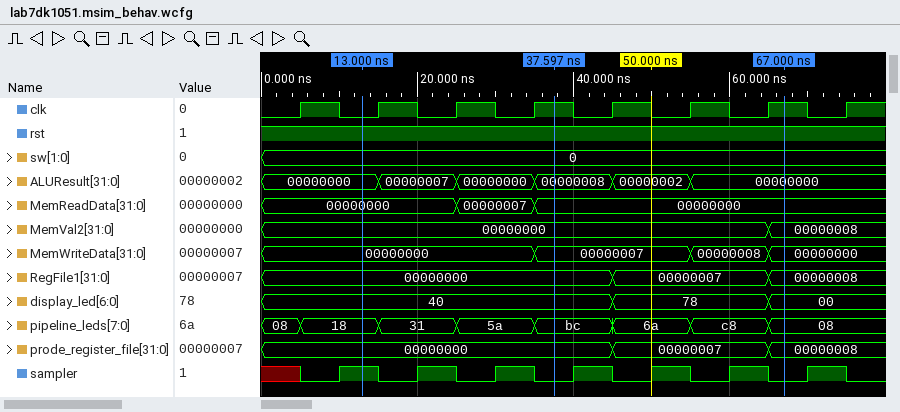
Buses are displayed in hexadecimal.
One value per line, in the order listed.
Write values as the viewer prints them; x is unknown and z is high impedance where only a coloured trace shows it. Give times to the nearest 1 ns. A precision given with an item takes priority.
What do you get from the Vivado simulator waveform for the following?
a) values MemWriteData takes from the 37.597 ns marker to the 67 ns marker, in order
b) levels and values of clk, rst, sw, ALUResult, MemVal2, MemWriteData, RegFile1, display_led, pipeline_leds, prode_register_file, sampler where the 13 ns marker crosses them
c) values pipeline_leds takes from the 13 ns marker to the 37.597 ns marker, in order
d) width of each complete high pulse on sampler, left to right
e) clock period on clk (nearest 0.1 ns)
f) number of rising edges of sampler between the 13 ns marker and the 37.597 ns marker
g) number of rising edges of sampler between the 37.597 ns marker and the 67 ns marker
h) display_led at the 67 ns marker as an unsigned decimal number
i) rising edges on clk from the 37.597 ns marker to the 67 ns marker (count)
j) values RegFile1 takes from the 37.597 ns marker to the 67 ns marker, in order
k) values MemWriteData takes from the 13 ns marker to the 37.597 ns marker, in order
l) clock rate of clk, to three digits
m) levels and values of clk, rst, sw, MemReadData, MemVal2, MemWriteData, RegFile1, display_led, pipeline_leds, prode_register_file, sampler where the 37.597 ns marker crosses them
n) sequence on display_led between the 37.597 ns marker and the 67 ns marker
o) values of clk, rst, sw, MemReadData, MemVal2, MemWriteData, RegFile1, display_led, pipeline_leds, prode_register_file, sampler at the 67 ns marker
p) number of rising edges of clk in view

00000007, 00000008, 00000000
clk=0, rst=1, sw=0, ALUResult=00000000, MemVal2=00000000, MemWriteData=00000000, RegFile1=00000000, display_led=40, pipeline_leds=18, prode_register_file=00000000, sampler=1
18, 31, 5a, bc
5 ns, 5 ns, 5 ns, 5 ns, 5 ns, 5 ns, 5 ns
10 ns
2
3
0
3
00000000, 00000007, 00000008
00000000, 00000007
100 MHz
clk=1, rst=1, sw=0, MemReadData=00000000, MemVal2=00000000, MemWriteData=00000007, RegFile1=00000000, display_led=40, pipeline_leds=bc, prode_register_file=00000000, sampler=0
40, 78, 00
clk=1, rst=1, sw=0, MemReadData=00000000, MemVal2=00000008, MemWriteData=00000000, RegFile1=00000008, display_led=00, pipeline_leds=08, prode_register_file=00000008, sampler=0
8
